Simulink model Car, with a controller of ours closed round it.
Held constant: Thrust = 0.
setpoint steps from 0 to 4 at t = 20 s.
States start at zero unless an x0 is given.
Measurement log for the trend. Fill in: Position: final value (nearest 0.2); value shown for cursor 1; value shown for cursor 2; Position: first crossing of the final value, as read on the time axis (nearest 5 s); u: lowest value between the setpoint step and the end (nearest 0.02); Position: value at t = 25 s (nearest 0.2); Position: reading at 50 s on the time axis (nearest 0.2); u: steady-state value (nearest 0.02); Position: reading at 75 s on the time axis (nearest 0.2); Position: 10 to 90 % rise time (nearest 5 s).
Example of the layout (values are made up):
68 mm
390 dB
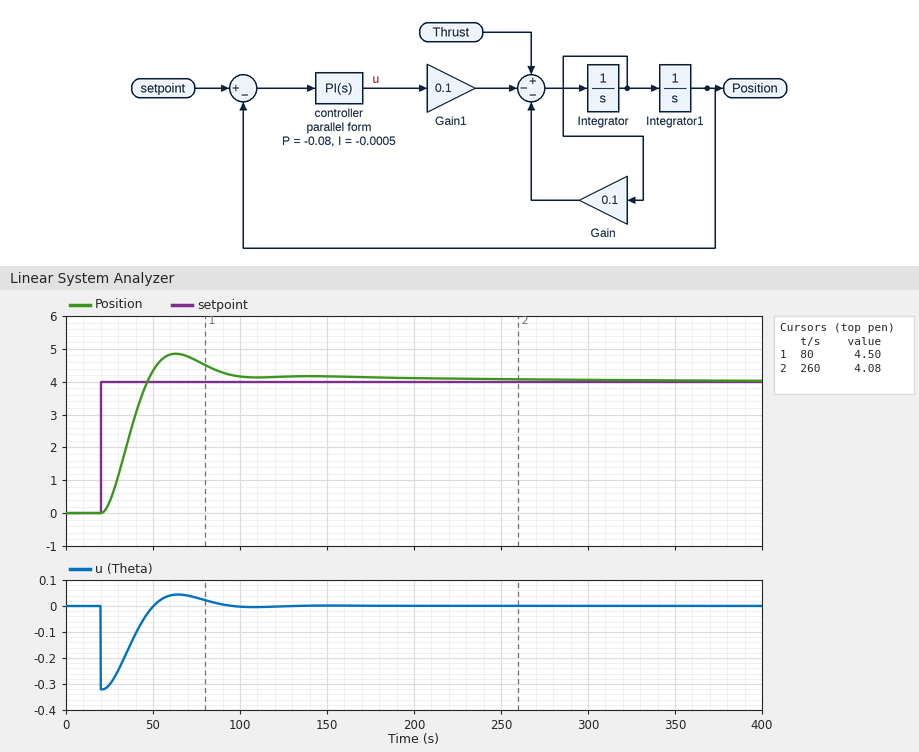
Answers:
4.0
4.50
4.08
45 s
-0.32
0.4
4.4
0.00
4.6
20 s
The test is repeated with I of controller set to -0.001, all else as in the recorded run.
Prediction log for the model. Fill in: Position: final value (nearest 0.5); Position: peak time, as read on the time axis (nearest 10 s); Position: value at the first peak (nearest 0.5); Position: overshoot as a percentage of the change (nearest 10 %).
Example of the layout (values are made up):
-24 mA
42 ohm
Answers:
4.0
60 s
5.0
30 %
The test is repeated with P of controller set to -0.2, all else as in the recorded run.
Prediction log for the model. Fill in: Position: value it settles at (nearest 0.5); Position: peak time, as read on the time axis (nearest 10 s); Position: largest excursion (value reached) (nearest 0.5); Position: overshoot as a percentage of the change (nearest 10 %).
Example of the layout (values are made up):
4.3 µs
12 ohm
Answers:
4.0
40 s
5.5
30 %
